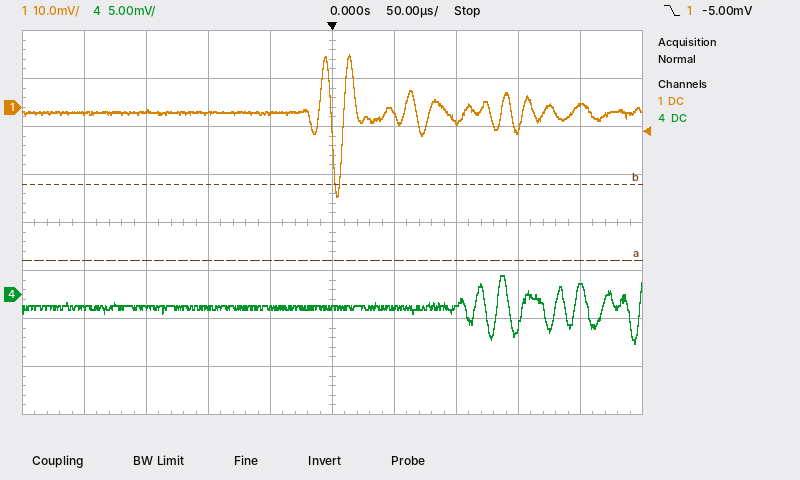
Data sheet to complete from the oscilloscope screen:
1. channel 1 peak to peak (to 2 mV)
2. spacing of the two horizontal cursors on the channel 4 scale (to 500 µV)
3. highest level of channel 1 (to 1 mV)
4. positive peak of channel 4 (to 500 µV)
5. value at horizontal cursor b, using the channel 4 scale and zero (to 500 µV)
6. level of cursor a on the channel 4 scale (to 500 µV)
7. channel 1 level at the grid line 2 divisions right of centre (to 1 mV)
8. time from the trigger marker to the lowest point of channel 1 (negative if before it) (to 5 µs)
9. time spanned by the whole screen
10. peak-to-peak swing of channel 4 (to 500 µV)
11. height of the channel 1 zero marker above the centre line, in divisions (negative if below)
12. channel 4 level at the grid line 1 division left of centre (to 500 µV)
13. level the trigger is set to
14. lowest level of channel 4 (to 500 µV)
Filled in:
30 mV
8.0 mV
11 mV
2.0 mV
11.5 mV
3.5 mV
-3 mV
+5 µs
500 µs
7.0 mV
+2.4 div
-1.5 mV
-5.00 mV
-5.0 mV
